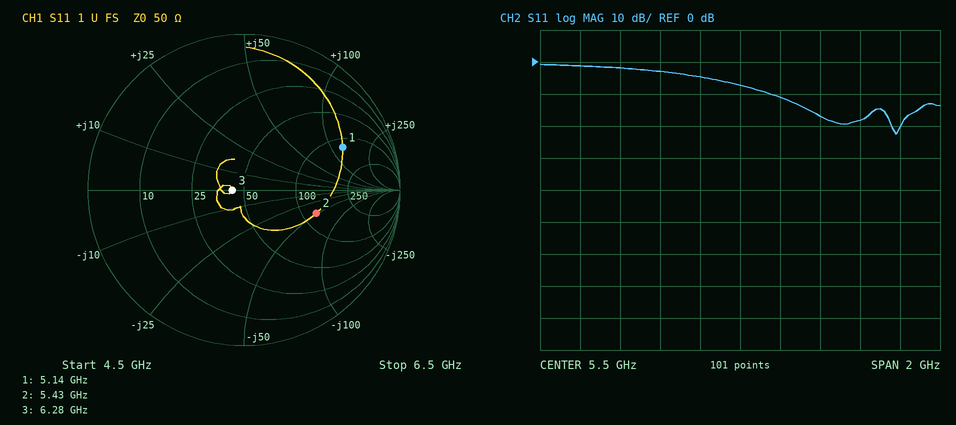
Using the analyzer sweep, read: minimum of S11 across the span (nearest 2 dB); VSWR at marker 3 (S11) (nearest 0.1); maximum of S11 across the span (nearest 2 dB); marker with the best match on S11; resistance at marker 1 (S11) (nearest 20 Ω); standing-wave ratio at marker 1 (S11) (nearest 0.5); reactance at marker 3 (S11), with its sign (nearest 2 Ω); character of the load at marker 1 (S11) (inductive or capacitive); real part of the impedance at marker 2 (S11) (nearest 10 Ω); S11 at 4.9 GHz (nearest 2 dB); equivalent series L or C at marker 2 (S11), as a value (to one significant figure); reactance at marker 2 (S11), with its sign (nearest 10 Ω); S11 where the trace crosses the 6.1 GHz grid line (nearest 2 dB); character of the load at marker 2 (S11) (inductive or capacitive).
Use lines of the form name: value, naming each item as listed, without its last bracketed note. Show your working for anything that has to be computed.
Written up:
minimum of S11 across the span: -22 dB
VSWR at marker 3 (S11): 1.2
maximum of S11 across the span: 0 dB
marker with the best match on S11: marker 3
resistance at marker 1 (S11): 120 Ω
standing-wave ratio at marker 1 (S11): 5.5
reactance at marker 3 (S11), with its sign: 0 Ω
character of the load at marker 1 (S11): inductive
real part of the impedance at marker 2 (S11): 120 Ω
S11 at 4.9 GHz: -2 dB
equivalent series L or C at marker 2 (S11), as a value: C = 1/(2π × 5.43 GHz × 50 Ω) ≈ 586 fF, so 600 fF to one significant figure
reactance at marker 2 (S11), with its sign: -50 Ω
S11 where the trace crosses the 6.1 GHz grid line: -18 dB
character of the load at marker 2 (S11): capacitive
